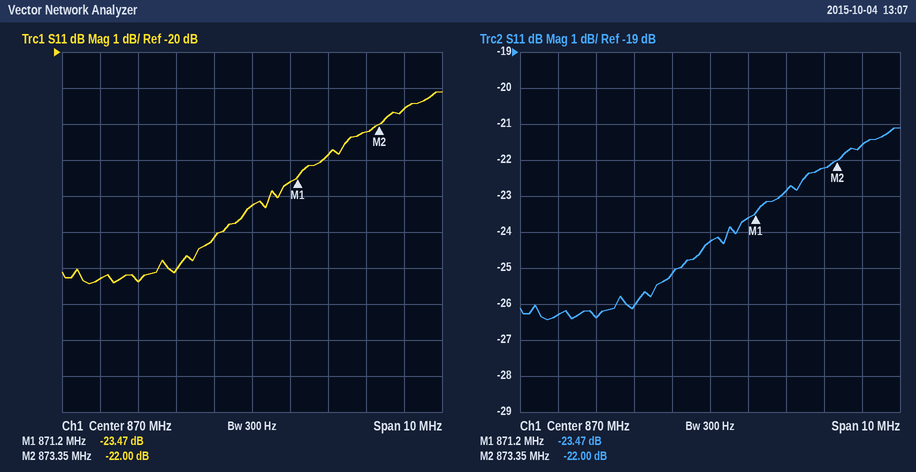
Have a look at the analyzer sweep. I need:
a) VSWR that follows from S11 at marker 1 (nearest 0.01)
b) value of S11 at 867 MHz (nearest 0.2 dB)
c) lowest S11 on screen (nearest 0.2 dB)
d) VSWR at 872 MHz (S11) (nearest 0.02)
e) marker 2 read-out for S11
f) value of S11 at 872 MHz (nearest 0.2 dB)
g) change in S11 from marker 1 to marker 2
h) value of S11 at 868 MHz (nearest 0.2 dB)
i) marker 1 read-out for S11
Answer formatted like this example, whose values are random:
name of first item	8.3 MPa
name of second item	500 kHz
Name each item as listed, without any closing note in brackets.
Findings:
VSWR that follows from S11 at marker 1	1.14
value of S11 at 867 MHz	-26.4 dB
lowest S11 on screen	-26.4 dB
VSWR at 872 MHz (S11)	1.16
marker 2 read-out for S11	-22.00 dB
value of S11 at 872 MHz	-22.8 dB
change in S11 from marker 1 to marker 2	1.47 dB
value of S11 at 868 MHz	-26.0 dB
marker 1 read-out for S11	-23.47 dB
